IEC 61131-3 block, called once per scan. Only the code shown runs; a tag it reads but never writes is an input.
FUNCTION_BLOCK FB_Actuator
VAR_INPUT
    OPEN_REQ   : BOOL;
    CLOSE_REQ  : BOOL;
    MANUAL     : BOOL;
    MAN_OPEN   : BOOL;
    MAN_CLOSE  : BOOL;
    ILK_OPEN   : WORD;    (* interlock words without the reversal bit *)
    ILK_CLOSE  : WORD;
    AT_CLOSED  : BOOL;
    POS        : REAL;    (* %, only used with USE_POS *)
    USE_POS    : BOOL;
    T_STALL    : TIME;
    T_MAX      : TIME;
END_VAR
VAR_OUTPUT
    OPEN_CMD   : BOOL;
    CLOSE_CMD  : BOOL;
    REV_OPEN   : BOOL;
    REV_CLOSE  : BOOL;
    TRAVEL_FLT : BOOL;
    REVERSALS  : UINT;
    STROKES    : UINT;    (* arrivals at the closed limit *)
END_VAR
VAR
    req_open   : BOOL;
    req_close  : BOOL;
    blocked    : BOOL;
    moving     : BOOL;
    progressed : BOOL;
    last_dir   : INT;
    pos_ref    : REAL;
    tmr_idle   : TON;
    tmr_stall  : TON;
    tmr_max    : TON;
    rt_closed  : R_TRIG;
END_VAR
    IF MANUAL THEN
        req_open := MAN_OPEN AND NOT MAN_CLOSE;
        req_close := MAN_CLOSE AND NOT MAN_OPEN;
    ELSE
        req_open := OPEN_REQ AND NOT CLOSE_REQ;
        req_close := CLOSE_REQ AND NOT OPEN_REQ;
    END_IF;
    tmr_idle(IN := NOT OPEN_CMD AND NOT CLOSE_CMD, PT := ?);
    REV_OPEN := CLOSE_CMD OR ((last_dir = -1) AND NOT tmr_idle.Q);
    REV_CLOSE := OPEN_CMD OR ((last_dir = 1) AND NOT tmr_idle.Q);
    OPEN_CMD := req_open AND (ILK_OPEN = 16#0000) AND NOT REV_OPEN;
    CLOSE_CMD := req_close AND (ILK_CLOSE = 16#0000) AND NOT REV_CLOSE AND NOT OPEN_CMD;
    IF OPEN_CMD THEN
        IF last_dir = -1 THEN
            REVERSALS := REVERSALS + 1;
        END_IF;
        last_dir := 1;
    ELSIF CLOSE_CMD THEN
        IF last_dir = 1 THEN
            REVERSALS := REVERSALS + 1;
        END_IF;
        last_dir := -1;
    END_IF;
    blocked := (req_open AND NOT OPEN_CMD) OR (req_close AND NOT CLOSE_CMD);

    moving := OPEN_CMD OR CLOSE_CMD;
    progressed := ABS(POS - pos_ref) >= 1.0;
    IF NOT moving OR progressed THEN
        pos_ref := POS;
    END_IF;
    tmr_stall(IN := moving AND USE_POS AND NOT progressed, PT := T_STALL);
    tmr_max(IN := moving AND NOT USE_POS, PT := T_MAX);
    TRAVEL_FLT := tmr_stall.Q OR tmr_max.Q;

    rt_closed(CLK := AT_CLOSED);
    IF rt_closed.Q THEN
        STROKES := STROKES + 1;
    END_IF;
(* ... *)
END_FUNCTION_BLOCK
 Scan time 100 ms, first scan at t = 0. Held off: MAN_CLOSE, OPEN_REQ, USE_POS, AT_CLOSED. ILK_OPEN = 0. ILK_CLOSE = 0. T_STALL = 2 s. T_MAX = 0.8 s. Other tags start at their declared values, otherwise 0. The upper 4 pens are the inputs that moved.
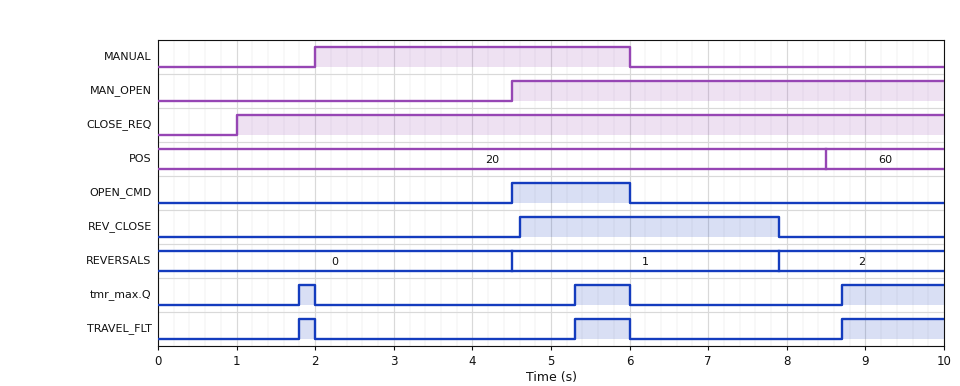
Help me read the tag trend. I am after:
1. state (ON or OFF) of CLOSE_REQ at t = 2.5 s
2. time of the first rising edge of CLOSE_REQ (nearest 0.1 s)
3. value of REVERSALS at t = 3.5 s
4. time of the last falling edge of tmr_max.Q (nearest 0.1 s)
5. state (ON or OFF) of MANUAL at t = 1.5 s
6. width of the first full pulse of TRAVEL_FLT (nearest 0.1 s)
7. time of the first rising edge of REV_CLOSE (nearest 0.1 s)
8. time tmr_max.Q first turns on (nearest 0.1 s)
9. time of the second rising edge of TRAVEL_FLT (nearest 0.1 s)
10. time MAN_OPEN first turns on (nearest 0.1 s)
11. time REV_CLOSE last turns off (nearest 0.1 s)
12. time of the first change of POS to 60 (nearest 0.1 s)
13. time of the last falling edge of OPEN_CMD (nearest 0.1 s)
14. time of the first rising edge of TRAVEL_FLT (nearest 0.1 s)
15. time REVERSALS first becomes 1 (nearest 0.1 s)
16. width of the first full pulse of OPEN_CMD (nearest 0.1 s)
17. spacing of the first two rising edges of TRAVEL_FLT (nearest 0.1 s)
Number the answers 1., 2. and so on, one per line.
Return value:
1. ON
2. 1.0 s
3. 0
4. 6.0 s
5. OFF
6. 0.2 s
7. 4.6 s
8. 1.8 s
9. 5.3 s
10. 4.5 s
11. 7.9 s
12. 8.5 s
13. 6.0 s
14. 1.8 s
15. 4.5 s
16. 1.5 s
17. 3.5 s
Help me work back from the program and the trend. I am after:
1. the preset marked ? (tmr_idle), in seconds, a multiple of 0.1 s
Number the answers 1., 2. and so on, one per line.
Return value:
1. 1.8 s
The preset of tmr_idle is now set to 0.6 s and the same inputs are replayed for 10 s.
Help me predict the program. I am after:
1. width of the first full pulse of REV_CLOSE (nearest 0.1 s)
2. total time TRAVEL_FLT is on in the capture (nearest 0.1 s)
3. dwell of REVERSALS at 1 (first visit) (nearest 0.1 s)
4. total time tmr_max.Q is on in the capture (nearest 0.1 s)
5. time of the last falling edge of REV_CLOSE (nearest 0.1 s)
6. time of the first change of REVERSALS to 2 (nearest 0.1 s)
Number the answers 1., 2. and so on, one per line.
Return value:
1. 2.1 s
2. 3.4 s
3. 2.2 s
4. 3.4 s
5. 6.7 s
6. 6.7 s
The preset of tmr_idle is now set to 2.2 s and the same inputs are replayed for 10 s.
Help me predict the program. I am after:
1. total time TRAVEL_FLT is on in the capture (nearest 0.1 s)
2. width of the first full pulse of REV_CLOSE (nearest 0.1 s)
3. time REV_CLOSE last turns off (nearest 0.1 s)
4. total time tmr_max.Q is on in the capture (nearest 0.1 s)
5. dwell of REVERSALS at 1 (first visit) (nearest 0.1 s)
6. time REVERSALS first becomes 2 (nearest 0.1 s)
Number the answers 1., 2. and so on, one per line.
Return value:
1. 1.8 s
2. 3.7 s
3. 8.3 s
4. 1.8 s
5. 3.8 s
6. 8.3 s
